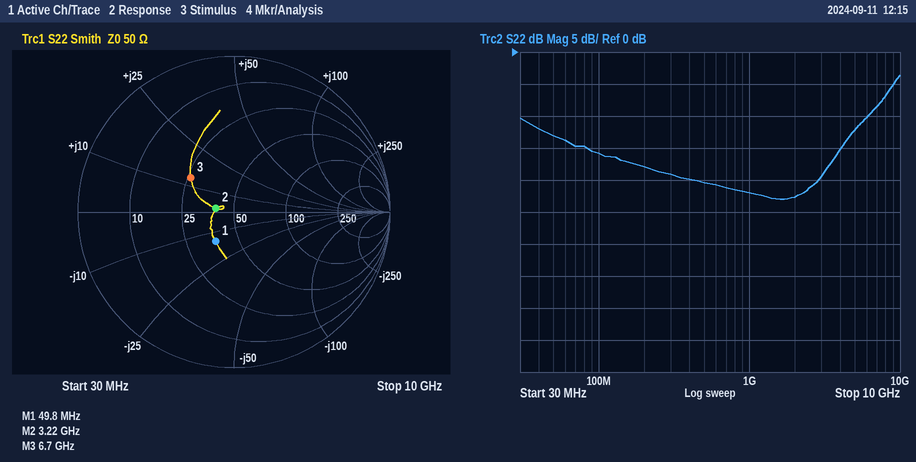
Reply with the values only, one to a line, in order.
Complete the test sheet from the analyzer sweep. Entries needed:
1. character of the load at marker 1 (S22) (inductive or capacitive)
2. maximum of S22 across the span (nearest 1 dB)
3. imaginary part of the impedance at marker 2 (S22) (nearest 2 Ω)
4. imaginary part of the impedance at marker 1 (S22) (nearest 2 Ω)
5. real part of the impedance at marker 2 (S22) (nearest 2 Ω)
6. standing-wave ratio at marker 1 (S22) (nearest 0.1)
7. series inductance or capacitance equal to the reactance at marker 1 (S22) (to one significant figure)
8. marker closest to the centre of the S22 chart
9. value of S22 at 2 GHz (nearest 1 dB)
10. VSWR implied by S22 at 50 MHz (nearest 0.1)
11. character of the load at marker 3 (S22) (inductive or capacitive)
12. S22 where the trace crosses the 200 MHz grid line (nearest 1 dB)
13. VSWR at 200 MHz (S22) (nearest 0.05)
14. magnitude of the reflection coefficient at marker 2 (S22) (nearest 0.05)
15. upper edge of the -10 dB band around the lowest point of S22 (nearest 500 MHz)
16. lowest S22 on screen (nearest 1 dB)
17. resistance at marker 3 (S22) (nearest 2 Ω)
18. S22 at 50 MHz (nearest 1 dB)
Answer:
capacitive
-4 dB
+2 Ω
-14 Ω
40 Ω
1.6
200 pF
marker 2
-23 dB
1.6
inductive
-18 dB
1.30
0.10
6.0 GHz
-23 dB
26 Ω
-13 dB
